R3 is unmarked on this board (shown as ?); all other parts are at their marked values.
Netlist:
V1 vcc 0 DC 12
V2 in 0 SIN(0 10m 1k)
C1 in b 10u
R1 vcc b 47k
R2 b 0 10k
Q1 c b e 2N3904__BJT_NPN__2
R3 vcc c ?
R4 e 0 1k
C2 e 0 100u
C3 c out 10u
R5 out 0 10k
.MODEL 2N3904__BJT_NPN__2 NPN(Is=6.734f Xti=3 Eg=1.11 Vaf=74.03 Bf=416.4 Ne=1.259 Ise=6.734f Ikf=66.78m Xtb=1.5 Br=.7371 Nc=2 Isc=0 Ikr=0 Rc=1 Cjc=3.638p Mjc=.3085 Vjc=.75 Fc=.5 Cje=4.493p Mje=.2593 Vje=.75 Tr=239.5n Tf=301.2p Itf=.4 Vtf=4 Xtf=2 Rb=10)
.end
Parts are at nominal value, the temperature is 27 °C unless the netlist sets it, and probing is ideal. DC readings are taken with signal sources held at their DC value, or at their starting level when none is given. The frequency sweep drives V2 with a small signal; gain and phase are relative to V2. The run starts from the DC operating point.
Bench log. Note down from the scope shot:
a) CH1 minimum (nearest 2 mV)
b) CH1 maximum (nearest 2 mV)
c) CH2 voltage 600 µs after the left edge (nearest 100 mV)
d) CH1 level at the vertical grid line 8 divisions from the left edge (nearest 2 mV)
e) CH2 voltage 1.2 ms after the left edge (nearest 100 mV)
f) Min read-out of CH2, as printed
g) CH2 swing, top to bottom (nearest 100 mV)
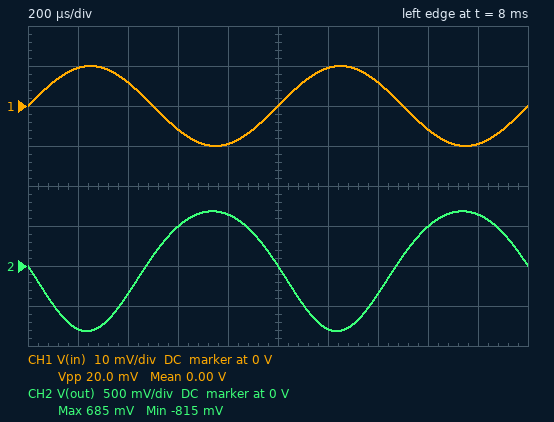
-10 mV
10 mV
500 mV
-6 mV
-800 mV
-815 mV
1.5 V
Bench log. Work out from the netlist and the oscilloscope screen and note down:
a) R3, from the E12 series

1.8 kΩ
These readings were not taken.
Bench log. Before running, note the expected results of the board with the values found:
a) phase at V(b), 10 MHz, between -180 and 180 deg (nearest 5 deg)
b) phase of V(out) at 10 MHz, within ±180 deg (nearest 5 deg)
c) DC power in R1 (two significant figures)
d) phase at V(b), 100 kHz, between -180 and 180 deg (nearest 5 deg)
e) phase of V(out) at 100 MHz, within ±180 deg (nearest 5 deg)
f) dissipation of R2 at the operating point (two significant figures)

0 deg
165 deg
2.1 mW
0 deg
105 deg
410 µW
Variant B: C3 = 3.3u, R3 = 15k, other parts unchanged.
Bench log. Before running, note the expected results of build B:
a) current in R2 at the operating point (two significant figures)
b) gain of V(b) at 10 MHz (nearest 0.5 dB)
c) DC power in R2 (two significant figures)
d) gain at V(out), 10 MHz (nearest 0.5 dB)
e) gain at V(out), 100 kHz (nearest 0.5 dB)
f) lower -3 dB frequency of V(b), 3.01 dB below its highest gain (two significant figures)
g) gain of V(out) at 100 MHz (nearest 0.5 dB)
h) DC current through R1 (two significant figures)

150 µA
0 dB
220 µW
0 dB
14.0 dB
280 Hz
-2.5 dB
220 µA
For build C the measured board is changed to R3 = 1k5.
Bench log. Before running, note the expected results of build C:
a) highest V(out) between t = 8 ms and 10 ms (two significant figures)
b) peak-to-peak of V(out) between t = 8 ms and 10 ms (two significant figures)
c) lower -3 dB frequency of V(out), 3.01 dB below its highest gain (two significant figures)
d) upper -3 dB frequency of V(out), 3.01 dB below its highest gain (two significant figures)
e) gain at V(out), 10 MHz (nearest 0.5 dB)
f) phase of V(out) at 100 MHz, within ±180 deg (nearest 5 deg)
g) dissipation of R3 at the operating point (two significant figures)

590 mV
1.3 V
87 Hz
47 MHz
36.0 dB
110 deg
2.7 mW
